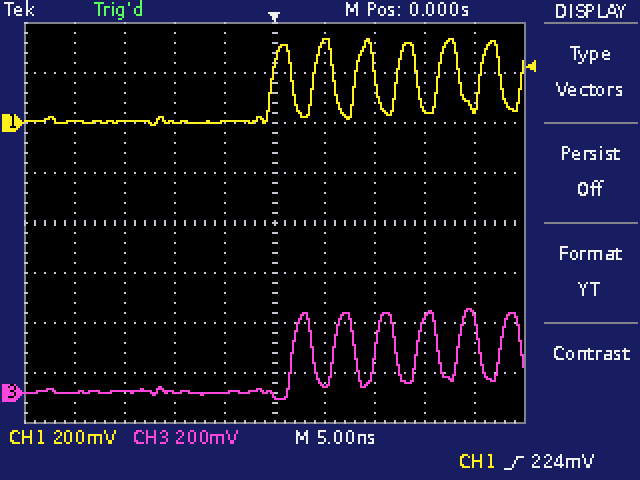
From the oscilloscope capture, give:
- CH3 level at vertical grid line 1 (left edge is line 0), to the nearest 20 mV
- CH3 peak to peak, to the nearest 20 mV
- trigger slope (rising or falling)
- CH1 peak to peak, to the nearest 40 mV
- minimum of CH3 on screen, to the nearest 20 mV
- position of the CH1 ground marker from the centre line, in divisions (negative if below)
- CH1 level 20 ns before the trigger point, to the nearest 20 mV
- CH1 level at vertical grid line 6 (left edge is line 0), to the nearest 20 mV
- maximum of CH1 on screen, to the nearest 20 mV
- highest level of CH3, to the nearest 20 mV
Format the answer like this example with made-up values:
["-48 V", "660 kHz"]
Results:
["0 mV", "360 mV", "rising", "360 mV", "-20 mV", "+2.0 div", "0 mV", "320 mV", "340 mV", "340 mV"]
